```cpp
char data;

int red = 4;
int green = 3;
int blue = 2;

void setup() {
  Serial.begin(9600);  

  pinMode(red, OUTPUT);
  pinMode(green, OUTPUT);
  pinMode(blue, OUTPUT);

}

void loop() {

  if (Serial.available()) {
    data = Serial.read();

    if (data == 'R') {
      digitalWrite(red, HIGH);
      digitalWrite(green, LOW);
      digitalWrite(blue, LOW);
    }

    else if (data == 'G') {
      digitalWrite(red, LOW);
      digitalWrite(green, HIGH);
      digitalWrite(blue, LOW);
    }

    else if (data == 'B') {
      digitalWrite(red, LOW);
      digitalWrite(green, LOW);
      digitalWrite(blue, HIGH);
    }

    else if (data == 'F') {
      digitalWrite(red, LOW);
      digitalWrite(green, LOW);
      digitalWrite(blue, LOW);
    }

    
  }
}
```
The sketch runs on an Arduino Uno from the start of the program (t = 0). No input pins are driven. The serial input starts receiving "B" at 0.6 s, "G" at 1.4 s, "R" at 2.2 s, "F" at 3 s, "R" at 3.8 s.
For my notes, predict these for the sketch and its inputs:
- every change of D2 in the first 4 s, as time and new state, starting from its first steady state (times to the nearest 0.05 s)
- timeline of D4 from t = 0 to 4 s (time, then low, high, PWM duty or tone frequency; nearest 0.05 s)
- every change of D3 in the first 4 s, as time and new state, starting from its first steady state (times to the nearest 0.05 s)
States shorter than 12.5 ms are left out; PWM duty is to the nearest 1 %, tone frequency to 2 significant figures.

0 s low; 0.6 s high; 1.4 s low
0 s low; 2.2 s high; 3 s low; 3.8 s high
0 s low; 1.4 s high; 2.2 s low
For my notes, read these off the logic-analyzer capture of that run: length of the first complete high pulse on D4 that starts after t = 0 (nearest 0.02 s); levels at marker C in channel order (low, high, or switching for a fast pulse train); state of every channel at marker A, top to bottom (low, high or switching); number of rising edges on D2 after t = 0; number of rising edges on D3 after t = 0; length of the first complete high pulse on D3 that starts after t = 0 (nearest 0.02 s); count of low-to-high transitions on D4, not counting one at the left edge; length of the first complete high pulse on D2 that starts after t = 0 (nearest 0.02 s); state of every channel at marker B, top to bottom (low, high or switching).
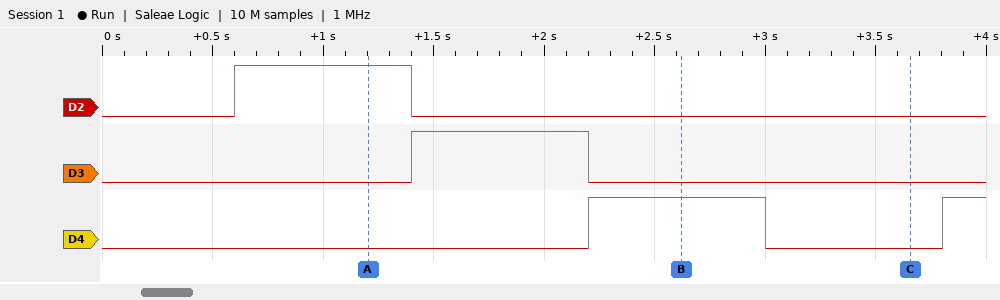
0.80 s
D2 low, D3 low, D4 low
D2 high, D3 low, D4 low
1
1
0.80 s
2
0.80 s
D2 low, D3 low, D4 high
